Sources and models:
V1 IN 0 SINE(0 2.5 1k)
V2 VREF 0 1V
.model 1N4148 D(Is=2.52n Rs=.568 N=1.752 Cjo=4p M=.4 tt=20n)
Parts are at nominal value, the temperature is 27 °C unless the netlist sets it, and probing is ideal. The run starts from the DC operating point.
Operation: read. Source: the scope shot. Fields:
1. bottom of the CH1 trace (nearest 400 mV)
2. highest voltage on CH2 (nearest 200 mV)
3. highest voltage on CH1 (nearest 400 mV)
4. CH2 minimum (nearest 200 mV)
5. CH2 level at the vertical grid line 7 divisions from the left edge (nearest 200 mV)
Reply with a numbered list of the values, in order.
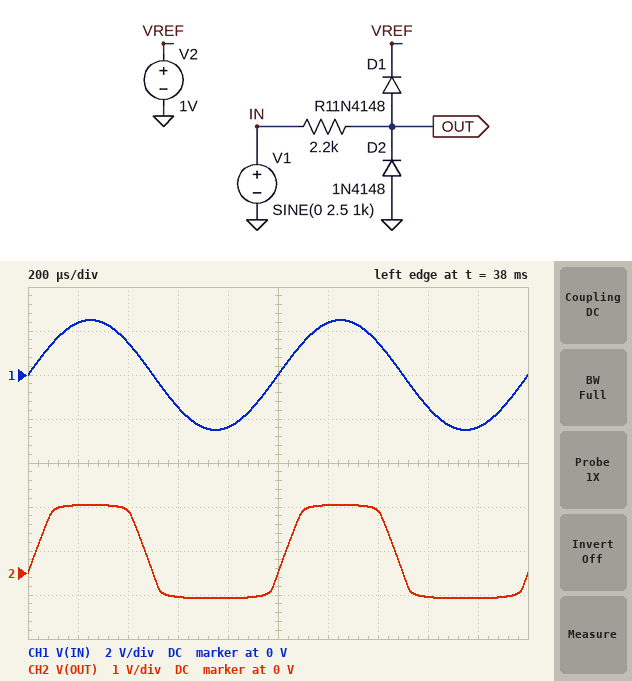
1. -2.4 V
2. 1.6 V
3. 2.4 V
4. -600 mV
5. 1.4 V
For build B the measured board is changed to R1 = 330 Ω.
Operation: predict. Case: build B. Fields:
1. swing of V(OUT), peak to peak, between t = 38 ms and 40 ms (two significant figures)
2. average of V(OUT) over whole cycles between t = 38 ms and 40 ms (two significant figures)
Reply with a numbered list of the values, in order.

1. 2.3 V
2. 340 mV
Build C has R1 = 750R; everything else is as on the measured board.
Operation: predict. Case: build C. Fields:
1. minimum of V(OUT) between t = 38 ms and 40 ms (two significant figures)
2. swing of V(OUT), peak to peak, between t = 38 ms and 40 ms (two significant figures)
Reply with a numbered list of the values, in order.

1. -630 mV
2. 2.2 V
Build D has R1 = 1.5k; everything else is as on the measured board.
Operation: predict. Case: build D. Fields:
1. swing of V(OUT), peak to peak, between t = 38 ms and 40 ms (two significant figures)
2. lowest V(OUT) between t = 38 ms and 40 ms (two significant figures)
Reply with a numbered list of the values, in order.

1. 2.2 V
2. -600 mV
